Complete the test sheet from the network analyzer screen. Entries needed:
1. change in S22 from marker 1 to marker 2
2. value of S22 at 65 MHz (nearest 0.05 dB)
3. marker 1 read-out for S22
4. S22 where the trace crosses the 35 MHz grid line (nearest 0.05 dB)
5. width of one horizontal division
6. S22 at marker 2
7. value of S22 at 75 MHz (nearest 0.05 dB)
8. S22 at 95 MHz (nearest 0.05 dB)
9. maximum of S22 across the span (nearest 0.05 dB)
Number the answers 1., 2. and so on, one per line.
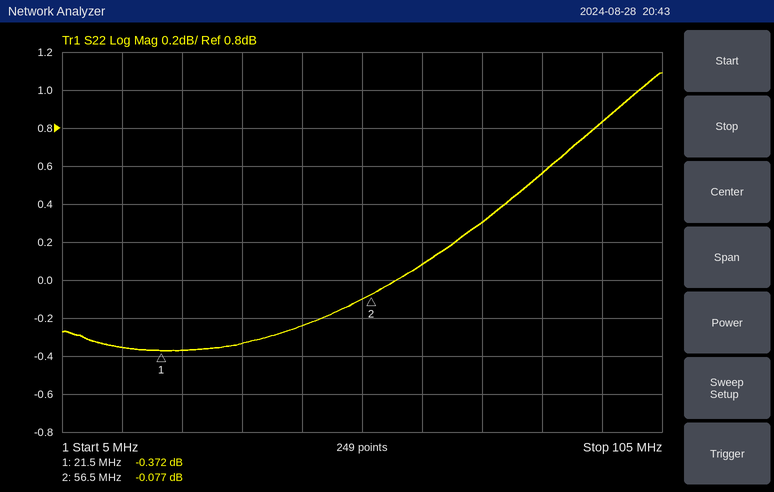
1. 0.295 dB
2. 0.10 dB
3. -0.372 dB
4. -0.35 dB
5. 10 MHz
6. -0.077 dB
7. 0.30 dB
8. 0.85 dB
9. 1.10 dB
